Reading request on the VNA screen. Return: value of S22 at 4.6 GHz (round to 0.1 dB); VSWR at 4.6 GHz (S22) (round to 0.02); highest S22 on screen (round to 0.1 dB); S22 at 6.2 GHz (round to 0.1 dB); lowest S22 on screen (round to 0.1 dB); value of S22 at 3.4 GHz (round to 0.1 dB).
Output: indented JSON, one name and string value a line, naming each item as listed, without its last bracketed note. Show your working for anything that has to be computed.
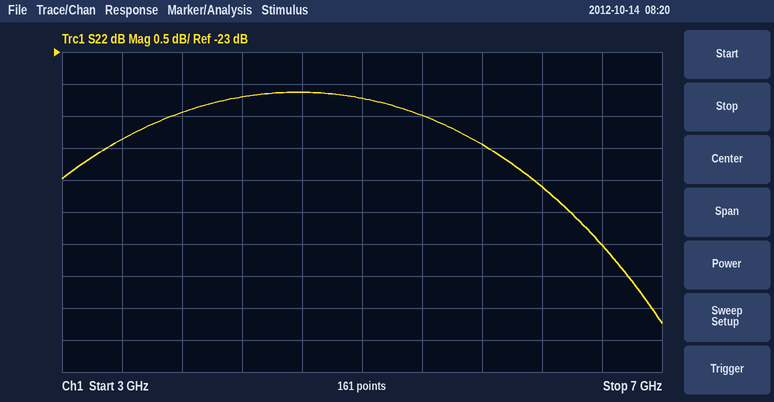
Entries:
{
  "value of S22 at 4.6 GHz": "-23.6 dB",
  "VSWR at 4.6 GHz (S22)": "|Γ| = 10^(-23.6/20) = 0.0661; VSWR = (1 + 0.0661)/(1 − 0.0661) ≈ 1.14",
  "highest S22 on screen": "-23.6 dB",
  "S22 at 6.2 GHz": "-25.1 dB",
  "lowest S22 on screen": "-27.2 dB",
  "value of S22 at 3.4 GHz": "-24.4 dB"
}
